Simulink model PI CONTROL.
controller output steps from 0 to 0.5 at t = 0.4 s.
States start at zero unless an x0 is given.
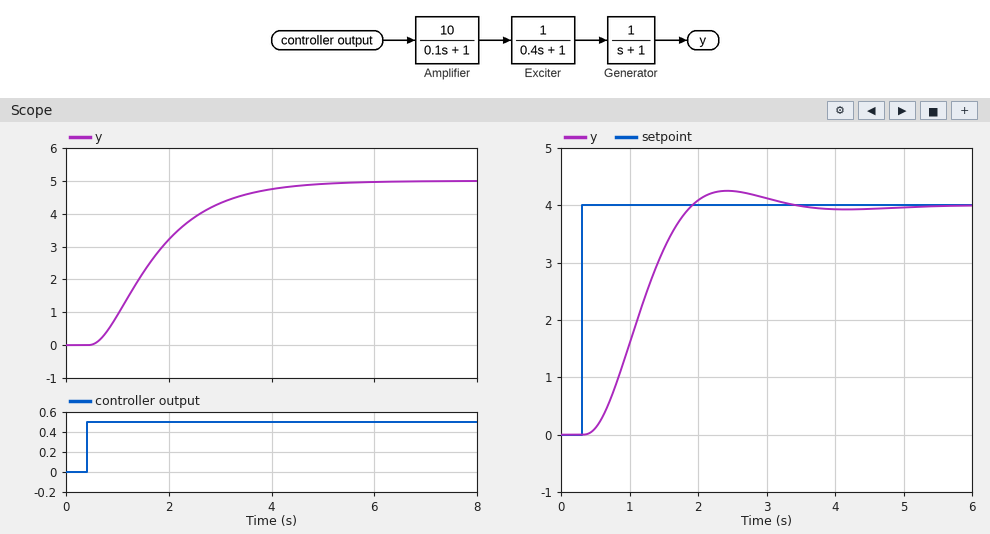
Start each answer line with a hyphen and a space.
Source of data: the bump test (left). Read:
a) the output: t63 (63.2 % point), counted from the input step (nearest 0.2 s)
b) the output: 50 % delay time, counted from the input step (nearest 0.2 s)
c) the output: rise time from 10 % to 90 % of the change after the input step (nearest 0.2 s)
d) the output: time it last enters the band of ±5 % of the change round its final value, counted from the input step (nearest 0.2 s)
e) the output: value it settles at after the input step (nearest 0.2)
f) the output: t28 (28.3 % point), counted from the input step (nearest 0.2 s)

- 1.6 s
- 1.2 s
- 2.4 s
- 3.6 s
- 5.0
- 0.8 s
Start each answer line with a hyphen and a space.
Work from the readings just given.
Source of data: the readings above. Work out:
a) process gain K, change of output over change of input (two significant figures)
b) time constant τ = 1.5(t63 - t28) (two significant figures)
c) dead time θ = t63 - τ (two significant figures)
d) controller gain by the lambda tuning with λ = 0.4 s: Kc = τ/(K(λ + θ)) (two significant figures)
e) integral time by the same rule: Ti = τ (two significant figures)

- 10
- 1.2 s
- 0.40 s
- 0.15
- 1.2 s
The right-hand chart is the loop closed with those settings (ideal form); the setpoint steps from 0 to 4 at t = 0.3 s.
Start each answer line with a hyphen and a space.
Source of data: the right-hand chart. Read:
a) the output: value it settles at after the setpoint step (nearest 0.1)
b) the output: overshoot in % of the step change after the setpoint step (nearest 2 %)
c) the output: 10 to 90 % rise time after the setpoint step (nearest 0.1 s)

- 4.0
- 6 %
- 1.0 s
